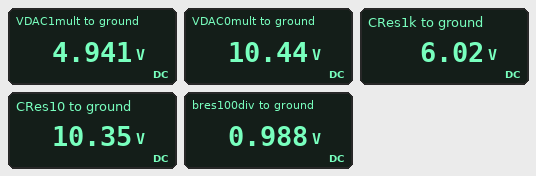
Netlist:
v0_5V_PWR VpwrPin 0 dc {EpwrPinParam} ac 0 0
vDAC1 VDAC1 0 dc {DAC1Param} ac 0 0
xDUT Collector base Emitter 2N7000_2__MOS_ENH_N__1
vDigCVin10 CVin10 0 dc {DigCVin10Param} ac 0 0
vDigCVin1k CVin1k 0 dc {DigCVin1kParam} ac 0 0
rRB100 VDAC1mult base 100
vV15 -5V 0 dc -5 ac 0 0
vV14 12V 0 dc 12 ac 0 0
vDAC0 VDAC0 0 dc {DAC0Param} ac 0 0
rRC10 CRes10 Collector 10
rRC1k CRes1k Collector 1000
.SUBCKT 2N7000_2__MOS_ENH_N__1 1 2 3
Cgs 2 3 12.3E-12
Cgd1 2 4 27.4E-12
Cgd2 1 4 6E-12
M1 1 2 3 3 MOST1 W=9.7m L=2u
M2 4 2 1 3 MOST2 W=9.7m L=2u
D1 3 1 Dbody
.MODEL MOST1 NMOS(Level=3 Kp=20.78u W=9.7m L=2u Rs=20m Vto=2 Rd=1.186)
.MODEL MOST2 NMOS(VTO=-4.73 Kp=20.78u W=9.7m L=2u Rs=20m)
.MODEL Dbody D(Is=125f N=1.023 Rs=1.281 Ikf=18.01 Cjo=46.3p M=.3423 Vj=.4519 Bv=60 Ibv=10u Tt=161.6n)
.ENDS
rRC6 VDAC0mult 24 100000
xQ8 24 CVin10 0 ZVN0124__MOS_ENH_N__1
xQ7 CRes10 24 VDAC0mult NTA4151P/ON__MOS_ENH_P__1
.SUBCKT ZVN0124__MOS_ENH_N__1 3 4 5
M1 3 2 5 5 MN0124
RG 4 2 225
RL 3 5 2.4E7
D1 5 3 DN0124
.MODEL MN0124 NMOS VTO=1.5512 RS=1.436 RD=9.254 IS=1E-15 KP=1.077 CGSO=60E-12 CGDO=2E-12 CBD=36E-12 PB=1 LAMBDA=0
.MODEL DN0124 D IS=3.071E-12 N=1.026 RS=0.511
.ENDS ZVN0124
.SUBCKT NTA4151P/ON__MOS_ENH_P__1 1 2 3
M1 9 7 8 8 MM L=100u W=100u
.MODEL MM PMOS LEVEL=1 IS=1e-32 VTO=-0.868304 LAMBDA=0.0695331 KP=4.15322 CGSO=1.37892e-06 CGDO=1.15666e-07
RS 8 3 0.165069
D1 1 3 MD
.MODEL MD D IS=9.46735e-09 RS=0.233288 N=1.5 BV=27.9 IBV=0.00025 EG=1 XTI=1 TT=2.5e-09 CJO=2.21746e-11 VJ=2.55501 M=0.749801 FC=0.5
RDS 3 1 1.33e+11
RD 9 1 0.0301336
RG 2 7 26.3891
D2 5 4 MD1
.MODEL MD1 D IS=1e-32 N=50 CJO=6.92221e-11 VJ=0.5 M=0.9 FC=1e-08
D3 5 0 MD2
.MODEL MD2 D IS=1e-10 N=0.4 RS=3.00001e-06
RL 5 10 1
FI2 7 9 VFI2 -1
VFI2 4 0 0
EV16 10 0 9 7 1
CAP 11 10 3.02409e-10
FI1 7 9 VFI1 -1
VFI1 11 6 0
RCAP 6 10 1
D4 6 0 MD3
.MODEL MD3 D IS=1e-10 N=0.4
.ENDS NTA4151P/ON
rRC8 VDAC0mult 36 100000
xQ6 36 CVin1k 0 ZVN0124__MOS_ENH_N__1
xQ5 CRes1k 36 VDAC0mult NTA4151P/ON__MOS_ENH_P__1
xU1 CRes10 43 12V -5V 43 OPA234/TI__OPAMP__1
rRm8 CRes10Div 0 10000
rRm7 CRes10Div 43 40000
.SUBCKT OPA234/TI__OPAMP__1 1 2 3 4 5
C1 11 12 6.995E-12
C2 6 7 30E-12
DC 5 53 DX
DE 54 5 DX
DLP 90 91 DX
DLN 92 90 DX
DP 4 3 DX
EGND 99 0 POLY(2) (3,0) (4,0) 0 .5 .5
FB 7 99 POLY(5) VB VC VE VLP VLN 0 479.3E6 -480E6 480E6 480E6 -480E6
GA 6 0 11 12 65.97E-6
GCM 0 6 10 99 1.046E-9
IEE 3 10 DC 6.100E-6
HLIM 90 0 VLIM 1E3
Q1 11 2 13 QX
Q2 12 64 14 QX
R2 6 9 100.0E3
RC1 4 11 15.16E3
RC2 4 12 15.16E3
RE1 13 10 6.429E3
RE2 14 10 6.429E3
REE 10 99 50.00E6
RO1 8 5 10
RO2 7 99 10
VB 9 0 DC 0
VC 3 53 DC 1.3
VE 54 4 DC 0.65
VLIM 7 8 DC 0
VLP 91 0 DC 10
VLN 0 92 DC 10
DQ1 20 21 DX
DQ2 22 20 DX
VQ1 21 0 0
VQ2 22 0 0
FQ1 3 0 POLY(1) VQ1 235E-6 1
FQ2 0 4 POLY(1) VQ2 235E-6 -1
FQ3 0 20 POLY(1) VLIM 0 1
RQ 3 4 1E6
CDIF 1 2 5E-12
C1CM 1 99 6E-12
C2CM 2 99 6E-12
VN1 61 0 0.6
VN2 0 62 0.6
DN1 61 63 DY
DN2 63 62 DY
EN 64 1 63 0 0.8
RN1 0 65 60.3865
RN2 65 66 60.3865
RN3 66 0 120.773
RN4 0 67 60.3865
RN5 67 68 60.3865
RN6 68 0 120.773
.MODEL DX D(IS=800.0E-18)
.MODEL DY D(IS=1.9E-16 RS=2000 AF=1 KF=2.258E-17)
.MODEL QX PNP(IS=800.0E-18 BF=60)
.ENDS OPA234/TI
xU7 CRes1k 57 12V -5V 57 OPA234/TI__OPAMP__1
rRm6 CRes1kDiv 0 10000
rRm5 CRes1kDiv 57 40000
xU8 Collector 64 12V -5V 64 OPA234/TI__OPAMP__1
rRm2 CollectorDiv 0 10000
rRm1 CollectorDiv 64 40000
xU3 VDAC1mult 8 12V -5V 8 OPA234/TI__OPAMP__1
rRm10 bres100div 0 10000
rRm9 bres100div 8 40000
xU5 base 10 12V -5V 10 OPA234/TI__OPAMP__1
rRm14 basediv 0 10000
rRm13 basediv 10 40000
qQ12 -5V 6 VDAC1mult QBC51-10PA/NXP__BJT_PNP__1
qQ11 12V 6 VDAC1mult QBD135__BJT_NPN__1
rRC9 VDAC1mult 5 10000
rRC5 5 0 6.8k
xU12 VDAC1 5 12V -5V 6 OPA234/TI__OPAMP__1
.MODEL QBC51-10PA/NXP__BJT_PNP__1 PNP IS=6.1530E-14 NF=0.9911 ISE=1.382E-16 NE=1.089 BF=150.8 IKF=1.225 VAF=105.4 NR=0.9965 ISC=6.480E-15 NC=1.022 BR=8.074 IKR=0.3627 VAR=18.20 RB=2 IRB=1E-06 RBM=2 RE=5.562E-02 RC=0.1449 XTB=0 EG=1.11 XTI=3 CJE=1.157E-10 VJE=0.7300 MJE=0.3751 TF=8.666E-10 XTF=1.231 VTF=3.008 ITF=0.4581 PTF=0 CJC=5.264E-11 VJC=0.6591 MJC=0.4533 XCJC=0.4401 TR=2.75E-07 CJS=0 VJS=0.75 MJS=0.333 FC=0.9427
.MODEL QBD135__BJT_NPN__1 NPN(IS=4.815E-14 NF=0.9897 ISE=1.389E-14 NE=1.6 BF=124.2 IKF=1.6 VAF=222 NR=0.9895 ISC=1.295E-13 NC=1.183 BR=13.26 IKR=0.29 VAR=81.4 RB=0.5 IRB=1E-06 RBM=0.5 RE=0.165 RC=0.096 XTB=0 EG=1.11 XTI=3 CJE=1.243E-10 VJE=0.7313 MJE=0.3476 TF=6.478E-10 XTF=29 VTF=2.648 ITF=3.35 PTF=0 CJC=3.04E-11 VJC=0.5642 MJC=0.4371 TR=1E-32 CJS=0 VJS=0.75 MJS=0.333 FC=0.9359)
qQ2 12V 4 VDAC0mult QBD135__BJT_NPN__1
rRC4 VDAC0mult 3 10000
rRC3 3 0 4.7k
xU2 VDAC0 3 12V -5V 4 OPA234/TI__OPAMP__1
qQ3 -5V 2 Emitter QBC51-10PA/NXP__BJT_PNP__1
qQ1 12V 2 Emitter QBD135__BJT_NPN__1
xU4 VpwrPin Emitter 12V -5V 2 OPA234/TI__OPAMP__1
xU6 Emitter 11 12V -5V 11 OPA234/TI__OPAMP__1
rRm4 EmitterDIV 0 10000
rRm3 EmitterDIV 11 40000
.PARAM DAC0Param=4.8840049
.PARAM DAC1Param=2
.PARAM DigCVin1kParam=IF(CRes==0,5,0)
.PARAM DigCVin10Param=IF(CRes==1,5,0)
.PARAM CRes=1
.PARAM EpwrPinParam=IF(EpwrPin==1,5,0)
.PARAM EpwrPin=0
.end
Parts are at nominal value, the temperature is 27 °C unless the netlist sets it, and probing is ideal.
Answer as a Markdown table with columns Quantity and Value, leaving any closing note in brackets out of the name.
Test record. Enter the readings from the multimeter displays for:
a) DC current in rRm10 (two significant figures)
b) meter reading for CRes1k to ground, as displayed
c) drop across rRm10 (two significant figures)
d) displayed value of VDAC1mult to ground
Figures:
| Quantity | Value |
|---|---|
| DC current in rRm10 | 99 µA |
| meter reading for CRes1k to ground, as displayed | 6.02 V |
| drop across rRm10 | 990 mV |
| displayed value of VDAC1mult to ground | 4.941 V |
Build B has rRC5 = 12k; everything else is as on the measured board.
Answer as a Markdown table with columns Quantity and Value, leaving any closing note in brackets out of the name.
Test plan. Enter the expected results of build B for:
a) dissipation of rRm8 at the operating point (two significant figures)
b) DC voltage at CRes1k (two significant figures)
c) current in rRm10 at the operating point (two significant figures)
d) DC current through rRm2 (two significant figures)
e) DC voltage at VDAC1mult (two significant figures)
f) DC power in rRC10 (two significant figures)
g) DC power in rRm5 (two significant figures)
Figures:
| Quantity | Value |
|---|---|
| dissipation of rRm8 at the operating point | 440 µW |
| DC voltage at CRes1k | 9.1 V |
| current in rRm10 at the operating point | 73 µA |
| DC current through rRm2 | 180 µA |
| DC voltage at VDAC1mult | 3.7 V |
| DC power in rRC10 | 190 mW |
| DC power in rRm5 | 1.3 mW |
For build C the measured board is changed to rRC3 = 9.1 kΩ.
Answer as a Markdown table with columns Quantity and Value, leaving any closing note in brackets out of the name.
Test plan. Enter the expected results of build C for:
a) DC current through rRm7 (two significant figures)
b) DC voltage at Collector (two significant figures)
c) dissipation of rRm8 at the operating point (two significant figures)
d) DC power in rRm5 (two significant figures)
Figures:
| Quantity | Value |
|---|---|
| DC current through rRm7 | 200 µA |
| DC voltage at Collector | 5.8 V |
| dissipation of rRm8 at the operating point | 410 µW |
| DC power in rRm5 | 540 µW |
